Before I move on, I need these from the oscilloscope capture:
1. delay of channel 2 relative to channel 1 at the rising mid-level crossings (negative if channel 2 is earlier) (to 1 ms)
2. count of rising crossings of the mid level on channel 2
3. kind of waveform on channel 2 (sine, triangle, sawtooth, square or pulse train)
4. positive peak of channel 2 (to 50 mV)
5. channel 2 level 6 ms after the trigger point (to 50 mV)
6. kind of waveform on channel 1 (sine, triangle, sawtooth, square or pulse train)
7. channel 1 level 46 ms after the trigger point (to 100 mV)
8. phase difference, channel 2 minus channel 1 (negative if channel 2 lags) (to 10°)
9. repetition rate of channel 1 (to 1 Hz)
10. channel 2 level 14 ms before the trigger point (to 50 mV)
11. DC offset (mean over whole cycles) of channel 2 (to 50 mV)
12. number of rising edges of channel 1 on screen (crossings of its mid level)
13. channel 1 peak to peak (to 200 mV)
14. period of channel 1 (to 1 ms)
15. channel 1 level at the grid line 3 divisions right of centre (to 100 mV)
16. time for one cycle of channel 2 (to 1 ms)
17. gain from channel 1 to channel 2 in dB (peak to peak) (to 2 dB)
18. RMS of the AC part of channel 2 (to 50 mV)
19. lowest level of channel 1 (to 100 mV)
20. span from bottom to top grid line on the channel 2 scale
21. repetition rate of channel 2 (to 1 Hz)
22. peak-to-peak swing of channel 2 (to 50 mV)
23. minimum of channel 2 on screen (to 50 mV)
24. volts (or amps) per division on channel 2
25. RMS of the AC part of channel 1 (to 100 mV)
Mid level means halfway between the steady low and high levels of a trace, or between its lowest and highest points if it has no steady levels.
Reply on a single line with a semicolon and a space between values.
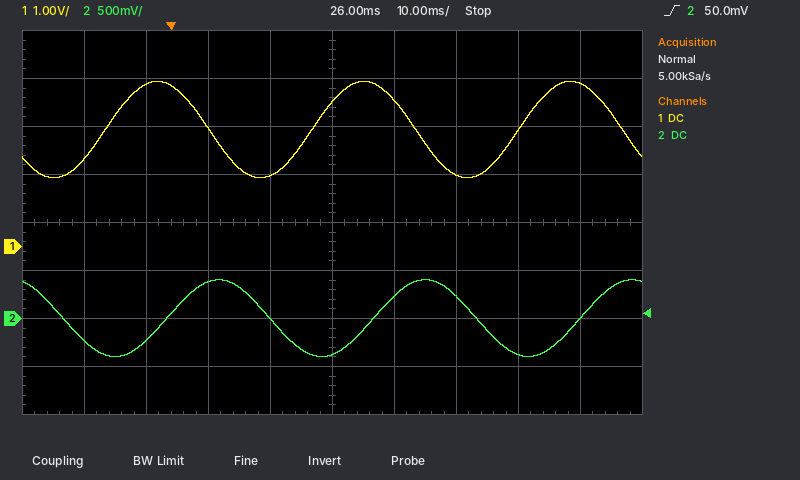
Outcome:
+10 ms; 3; sine; 400 mV; 400 mV; sine; 1.5 V; -110°; 30 Hz; -250 mV; 0 mV; 3; 2.0 V; 33 ms; 2.4 V; 33 ms; -8 dB; 300 mV; 1.4 V; 4 V; 30 Hz; 800 mV; -400 mV; 500 mV; 700 mV
